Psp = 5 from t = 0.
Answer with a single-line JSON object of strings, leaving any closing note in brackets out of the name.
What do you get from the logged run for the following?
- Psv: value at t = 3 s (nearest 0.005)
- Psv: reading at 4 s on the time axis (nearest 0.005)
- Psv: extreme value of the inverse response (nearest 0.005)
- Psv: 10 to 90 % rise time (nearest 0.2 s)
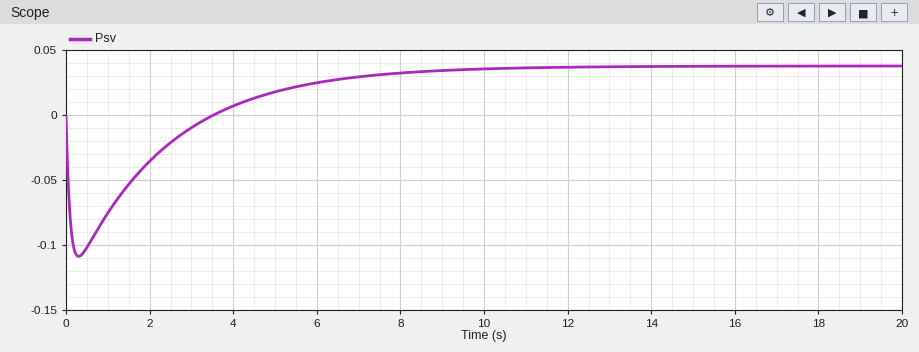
{"Psv: value at t = 3 s": "-0.010", "Psv: reading at 4 s on the time axis": "0.005", "Psv: extreme value of the inverse response": "-0.110", "Psv: 10 to 90 % rise time": "5.0 s"}
